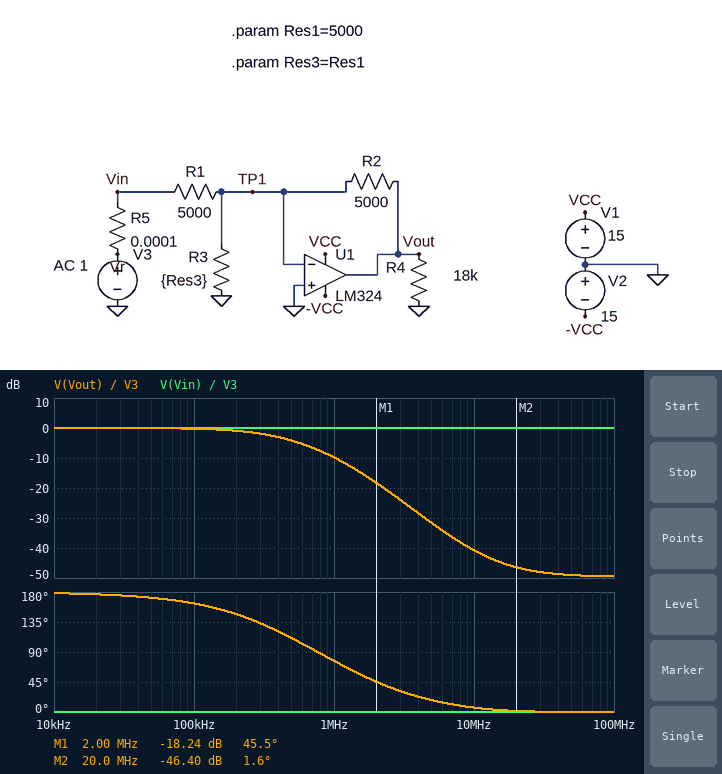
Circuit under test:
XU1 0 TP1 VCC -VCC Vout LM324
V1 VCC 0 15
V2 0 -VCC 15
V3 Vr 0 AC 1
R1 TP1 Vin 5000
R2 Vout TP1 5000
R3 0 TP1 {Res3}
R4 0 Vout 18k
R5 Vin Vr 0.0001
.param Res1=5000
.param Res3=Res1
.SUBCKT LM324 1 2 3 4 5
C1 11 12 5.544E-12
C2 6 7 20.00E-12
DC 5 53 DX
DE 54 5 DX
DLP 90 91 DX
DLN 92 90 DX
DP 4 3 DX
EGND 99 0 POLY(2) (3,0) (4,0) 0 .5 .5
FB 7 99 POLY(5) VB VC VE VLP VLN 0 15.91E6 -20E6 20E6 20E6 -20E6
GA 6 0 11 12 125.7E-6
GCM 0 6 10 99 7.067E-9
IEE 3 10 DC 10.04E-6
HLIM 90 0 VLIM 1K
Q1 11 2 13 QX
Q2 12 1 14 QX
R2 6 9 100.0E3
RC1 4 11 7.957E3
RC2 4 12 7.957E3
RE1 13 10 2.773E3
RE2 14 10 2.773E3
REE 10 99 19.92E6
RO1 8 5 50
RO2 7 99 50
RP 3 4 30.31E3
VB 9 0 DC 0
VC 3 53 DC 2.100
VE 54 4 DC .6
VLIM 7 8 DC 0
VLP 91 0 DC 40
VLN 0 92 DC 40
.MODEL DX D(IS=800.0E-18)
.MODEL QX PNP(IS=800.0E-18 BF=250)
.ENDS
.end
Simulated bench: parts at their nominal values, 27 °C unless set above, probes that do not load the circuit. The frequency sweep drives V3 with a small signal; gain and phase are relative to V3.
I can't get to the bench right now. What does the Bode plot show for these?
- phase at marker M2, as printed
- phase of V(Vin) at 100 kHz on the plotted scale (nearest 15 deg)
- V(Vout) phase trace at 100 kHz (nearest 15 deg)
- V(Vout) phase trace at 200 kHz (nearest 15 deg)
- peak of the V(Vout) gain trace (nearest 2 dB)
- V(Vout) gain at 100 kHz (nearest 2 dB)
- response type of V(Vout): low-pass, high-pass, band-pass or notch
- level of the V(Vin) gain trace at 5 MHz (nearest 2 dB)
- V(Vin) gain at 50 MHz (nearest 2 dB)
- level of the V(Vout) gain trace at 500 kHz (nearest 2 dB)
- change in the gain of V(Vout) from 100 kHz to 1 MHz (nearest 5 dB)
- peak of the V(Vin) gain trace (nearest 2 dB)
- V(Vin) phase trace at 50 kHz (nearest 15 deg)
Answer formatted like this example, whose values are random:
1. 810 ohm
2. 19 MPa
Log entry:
1. 1.6 deg
2. 0 deg
3. 165 deg
4. 150 deg
5. 0 dB
6. 0 dB
7. low-pass
8. 0 dB
9. 0 dB
10. -4 dB
11. -10 dB
12. 0 dB
13. 0 deg
